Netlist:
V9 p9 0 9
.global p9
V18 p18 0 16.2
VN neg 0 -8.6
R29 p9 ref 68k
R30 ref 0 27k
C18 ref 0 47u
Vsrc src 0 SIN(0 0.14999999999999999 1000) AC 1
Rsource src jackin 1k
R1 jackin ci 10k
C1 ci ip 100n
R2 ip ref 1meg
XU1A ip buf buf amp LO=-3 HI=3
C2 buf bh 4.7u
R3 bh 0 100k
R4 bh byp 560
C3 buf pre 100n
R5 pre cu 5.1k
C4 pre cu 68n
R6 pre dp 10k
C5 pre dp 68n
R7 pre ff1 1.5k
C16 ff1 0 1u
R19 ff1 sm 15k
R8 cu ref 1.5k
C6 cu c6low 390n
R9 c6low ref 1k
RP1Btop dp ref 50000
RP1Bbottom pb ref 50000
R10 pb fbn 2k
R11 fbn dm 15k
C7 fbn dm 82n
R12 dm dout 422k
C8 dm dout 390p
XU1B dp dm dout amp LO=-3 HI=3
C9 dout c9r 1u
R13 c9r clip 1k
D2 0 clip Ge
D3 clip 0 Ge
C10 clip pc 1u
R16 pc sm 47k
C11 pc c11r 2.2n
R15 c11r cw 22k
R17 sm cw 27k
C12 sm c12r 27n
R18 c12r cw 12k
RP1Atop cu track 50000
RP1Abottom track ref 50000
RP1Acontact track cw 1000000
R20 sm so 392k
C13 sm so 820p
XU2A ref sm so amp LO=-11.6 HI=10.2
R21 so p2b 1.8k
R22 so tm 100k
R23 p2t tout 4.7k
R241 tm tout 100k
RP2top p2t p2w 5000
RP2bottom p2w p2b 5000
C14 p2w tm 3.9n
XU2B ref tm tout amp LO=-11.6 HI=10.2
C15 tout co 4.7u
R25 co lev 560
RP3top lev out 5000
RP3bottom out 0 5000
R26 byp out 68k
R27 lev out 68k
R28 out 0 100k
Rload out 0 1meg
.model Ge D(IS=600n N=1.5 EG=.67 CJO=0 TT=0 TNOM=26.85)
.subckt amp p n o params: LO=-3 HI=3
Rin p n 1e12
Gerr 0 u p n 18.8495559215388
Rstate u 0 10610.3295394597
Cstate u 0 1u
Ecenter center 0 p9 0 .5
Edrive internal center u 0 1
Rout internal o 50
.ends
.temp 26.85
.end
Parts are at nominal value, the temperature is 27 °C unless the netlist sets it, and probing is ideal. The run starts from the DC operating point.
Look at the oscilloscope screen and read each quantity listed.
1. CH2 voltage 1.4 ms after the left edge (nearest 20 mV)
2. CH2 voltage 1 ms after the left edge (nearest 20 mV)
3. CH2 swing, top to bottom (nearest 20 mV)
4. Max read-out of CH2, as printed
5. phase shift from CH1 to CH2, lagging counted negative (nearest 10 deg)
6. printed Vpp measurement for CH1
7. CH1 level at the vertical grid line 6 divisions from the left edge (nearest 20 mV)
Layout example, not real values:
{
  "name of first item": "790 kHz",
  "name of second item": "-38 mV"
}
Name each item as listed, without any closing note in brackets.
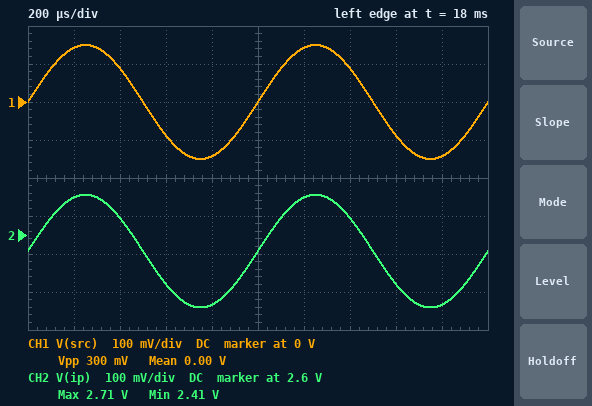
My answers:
{
  "CH2 voltage 1.4 ms after the left edge": "2.64 V",
  "CH2 voltage 1 ms after the left edge": "2.56 V",
  "CH2 swing, top to bottom": "300 mV",
  "Max read-out of CH2, as printed": "2.71 V",
  "phase shift from CH1 to CH2, lagging counted negative": "0 deg",
  "printed Vpp measurement for CH1": "300 mV",
  "CH1 level at the vertical grid line 6 divisions from the left edge": "140 mV"
}
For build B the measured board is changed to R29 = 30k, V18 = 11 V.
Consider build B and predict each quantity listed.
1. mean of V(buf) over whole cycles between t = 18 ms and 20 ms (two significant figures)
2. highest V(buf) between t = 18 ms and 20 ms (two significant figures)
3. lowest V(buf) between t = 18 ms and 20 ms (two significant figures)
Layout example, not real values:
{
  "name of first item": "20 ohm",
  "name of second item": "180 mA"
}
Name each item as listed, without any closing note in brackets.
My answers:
{
  "mean of V(buf) over whole cycles between t = 18 ms and 20 ms": "4.3 V",
  "highest V(buf) between t = 18 ms and 20 ms": "4.4 V",
  "lowest V(buf) between t = 18 ms and 20 ms": "4.1 V"
}
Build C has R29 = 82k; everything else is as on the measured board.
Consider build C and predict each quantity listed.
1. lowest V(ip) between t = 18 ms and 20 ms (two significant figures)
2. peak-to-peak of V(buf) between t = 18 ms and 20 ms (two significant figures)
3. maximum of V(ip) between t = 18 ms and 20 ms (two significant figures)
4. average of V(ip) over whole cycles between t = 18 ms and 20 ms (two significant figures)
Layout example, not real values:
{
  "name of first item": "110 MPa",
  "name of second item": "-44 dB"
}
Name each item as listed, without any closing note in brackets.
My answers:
{
  "lowest V(ip) between t = 18 ms and 20 ms": "2.1 V",
  "peak-to-peak of V(buf) between t = 18 ms and 20 ms": "300 mV",
  "maximum of V(ip) between t = 18 ms and 20 ms": "2.4 V",
  "average of V(ip) over whole cycles between t = 18 ms and 20 ms": "2.2 V"
}
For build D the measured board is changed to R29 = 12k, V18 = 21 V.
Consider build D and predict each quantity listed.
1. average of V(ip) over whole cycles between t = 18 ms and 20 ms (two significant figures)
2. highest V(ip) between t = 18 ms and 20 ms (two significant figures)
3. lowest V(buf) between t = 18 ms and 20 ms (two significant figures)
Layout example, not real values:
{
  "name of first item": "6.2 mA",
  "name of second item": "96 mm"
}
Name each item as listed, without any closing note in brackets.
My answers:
{
  "average of V(ip) over whole cycles between t = 18 ms and 20 ms": "6.2 V",
  "highest V(ip) between t = 18 ms and 20 ms": "6.4 V",
  "lowest V(buf) between t = 18 ms and 20 ms": "6.1 V"
}
